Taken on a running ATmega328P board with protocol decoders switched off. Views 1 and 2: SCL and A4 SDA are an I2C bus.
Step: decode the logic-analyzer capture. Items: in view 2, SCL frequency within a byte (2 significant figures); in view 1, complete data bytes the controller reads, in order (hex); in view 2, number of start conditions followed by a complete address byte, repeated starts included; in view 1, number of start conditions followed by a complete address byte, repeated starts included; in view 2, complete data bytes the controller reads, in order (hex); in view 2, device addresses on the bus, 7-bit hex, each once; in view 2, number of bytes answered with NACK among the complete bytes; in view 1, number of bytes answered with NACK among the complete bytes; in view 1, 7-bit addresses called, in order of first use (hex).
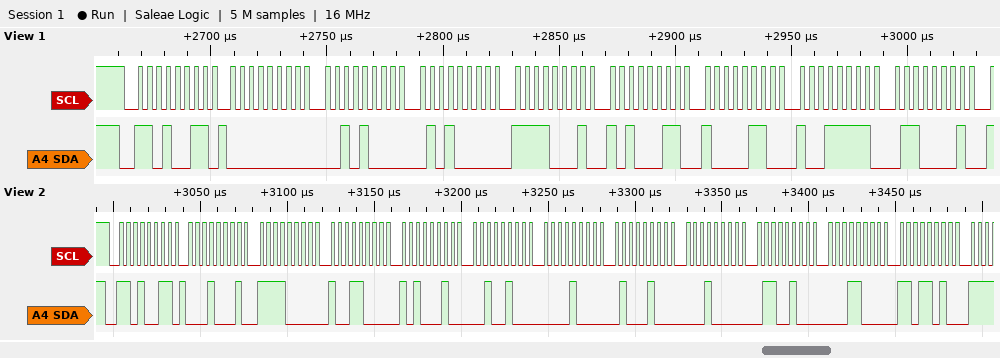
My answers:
250 kHz
00 28 50 F1 A3 86 9F 61
1
1
11 F0 98 A2 24 08 44 10 64 18 DA
0x69
0
0
0x69
